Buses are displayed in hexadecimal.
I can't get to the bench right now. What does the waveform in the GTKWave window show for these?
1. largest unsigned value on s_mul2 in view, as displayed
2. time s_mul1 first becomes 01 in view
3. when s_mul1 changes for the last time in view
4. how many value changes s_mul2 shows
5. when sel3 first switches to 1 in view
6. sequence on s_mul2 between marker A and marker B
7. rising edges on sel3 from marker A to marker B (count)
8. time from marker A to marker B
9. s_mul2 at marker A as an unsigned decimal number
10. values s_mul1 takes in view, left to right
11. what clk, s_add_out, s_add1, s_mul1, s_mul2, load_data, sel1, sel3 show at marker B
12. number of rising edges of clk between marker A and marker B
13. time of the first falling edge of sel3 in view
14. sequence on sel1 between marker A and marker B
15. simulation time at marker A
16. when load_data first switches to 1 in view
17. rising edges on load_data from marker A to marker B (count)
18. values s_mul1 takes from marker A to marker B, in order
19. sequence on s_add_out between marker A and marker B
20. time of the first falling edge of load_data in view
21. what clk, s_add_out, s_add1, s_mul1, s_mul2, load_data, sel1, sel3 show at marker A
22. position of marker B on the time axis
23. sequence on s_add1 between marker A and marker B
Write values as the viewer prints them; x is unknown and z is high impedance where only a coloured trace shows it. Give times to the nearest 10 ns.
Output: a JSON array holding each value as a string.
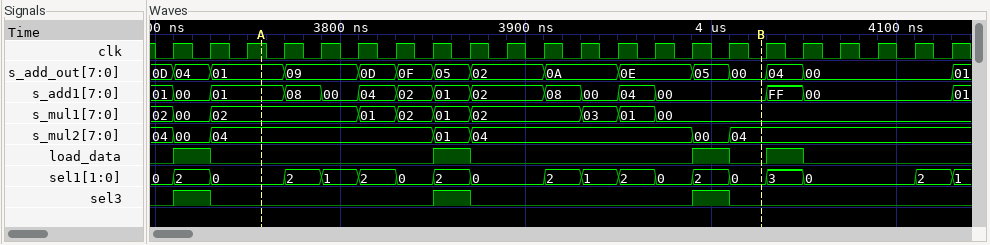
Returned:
["04", "3810 ns", "3970 ns", "6", "3710 ns", "04, 01, 04, 00, 04", "2", "270 ns", "4", "02, 00, 02, 01, 02, 01, 02, 03, 01, 00", "clk=0, s_add_out=00, s_add1=00, s_mul1=00, s_mul2=04, load_data=0, sel1=0, sel3=0", "13", "3730 ns", "0, 2, 1, 2, 0, 2, 0, 2, 1, 2, 0, 2, 0", "3760 ns", "3710 ns", "2", "02, 01, 02, 01, 02, 03, 01, 00", "01, 09, 0D, 0F, 05, 02, 0A, 0E, 05, 00", "3730 ns", "clk=1, s_add_out=01, s_add1=01, s_mul1=02, s_mul2=04, load_data=0, sel1=0, sel3=0", "4030 ns", "01, 08, 00, 04, 02, 01, 02, 08, 00, 04, 00"]
